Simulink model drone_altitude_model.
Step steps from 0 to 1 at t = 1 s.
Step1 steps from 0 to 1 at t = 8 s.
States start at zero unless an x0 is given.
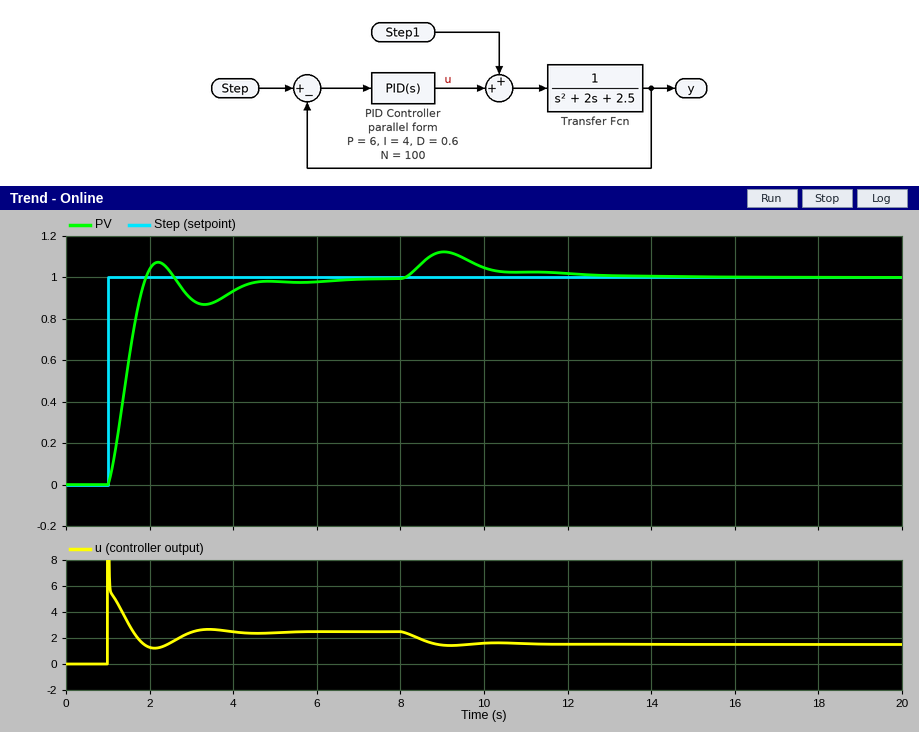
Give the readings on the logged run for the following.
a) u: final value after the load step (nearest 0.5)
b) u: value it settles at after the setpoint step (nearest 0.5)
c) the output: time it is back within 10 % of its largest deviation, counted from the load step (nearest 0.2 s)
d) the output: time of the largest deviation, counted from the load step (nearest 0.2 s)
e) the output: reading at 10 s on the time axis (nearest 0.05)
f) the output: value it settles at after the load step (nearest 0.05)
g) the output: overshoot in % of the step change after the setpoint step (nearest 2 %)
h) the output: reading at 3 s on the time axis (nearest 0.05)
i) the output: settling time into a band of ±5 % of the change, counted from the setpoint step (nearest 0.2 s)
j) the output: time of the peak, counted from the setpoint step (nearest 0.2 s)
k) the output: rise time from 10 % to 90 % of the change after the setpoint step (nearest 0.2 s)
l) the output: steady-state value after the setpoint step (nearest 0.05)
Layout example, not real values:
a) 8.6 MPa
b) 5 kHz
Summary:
a) 1.5
b) 2.5
c) 4.4 s
d) 1.0 s
e) 1.05
f) 1.00
g) 8 %
h) 0.90
i) 3.2 s
j) 1.2 s
k) 0.6 s
l) 1.00
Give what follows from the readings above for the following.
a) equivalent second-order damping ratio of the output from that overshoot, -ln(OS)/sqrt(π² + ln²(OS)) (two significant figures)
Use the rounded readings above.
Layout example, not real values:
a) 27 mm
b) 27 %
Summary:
a) 0.63
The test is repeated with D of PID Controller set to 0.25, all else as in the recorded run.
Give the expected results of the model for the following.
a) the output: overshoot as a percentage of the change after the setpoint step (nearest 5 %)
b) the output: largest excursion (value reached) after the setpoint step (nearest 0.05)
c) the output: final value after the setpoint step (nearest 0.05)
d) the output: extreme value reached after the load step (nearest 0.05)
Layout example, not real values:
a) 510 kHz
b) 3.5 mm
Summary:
a) 15 %
b) 1.15
c) 1.00
d) 1.15
